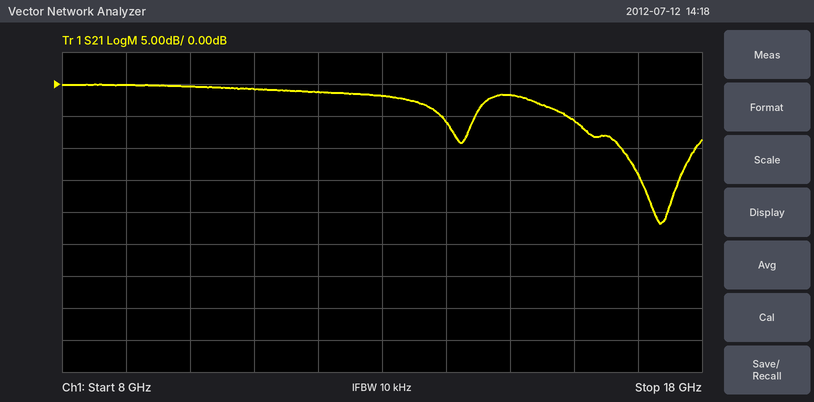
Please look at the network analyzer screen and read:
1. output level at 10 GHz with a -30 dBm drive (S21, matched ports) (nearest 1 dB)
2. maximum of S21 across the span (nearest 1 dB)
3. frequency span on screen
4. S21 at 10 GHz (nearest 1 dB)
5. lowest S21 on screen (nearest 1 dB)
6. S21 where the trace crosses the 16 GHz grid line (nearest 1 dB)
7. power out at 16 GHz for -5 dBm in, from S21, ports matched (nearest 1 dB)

-30 dBm
0 dB
10 GHz
0 dB
-22 dB
-6 dB
-11 dBm
